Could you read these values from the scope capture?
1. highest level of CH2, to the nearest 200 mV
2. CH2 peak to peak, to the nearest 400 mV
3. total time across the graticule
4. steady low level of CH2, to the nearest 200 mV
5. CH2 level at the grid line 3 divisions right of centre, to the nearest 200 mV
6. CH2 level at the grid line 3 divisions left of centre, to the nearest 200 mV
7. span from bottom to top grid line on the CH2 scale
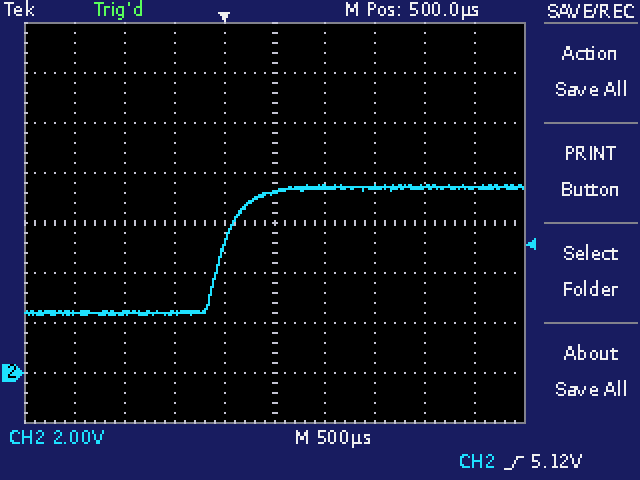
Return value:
7.6 V
5.2 V
5 ms
2.4 V
7.4 V
2.4 V
16 V
